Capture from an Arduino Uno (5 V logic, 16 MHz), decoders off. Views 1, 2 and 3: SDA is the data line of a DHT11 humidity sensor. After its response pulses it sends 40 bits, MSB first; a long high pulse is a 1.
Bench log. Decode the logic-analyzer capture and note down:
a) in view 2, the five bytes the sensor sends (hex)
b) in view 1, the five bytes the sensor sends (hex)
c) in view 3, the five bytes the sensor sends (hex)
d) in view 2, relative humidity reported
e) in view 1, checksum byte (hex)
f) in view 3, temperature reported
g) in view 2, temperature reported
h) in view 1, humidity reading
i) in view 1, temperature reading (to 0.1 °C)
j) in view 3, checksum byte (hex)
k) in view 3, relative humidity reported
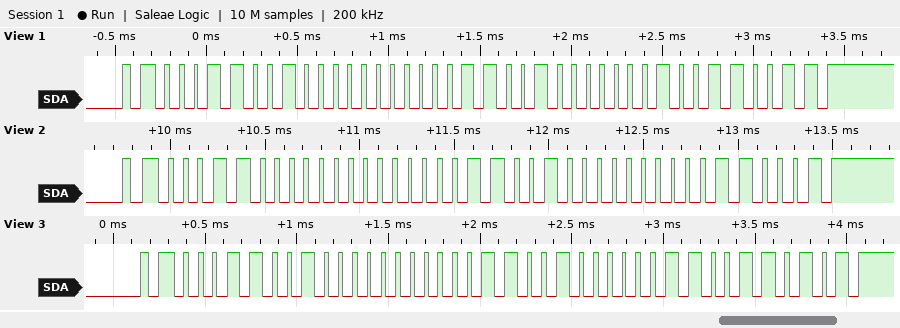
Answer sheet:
18 00 19 00 31
19 00 19 01 33
19 00 19 03 35
24 %
0x33
25.3 °C
25.0 °C
25 %
25.1 °C
0x35
25 %
